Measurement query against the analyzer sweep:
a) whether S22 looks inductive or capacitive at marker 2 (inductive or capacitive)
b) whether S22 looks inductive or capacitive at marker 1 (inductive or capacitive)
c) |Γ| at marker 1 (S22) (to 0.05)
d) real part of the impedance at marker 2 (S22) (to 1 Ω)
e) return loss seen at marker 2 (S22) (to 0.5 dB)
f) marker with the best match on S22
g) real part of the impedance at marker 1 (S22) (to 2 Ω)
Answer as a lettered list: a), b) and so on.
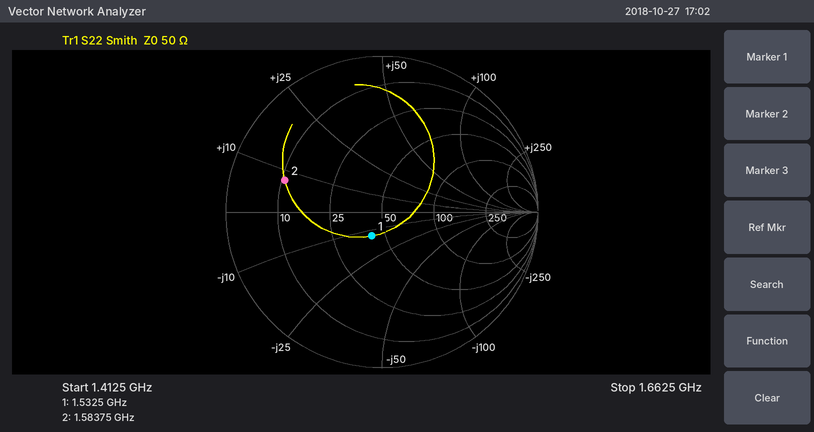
a) inductive
b) capacitive
c) 0.15
d) 11 Ω
e) 3.5 dB
f) marker 1
g) 42 Ω
